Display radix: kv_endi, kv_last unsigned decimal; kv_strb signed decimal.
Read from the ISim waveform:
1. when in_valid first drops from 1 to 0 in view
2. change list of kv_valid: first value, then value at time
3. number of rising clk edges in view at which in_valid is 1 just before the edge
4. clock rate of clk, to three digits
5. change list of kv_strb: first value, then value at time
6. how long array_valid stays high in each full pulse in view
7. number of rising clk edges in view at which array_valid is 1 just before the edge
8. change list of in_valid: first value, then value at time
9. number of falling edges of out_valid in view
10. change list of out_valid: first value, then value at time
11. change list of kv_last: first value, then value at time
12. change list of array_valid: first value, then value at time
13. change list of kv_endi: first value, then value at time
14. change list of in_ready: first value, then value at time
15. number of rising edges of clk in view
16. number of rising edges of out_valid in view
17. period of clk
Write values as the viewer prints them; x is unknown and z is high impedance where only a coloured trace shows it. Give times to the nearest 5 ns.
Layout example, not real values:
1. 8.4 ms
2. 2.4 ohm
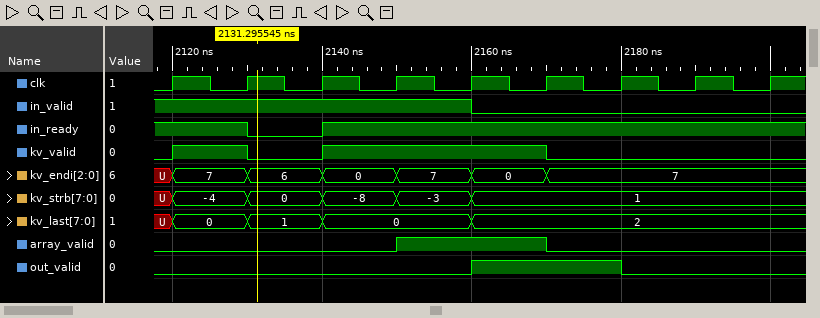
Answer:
1. 2160 ns
2. 0, 1 at 2120 ns, 0 at 2130 ns, 1 at 2140 ns, 0 at 2170 ns
3. 5
4. 100 MHz
5. U, -4 at 2120 ns, 0 at 2130 ns, -8 at 2140 ns, -3 at 2150 ns, 1 at 2160 ns
6. 20 ns
7. 2
8. 1, 0 at 2160 ns
9. 1
10. 0, 1 at 2160 ns, 0 at 2180 ns
11. U, 0 at 2120 ns, 1 at 2130 ns, 0 at 2140 ns, 2 at 2160 ns
12. 0, 1 at 2150 ns, 0 at 2170 ns
13. U, 7 at 2120 ns, 6 at 2130 ns, 0 at 2140 ns, 7 at 2150 ns, 0 at 2160 ns, 7 at 2170 ns
14. 1, 0 at 2130 ns, 1 at 2140 ns
15. 9
16. 1
17. 10 ns
